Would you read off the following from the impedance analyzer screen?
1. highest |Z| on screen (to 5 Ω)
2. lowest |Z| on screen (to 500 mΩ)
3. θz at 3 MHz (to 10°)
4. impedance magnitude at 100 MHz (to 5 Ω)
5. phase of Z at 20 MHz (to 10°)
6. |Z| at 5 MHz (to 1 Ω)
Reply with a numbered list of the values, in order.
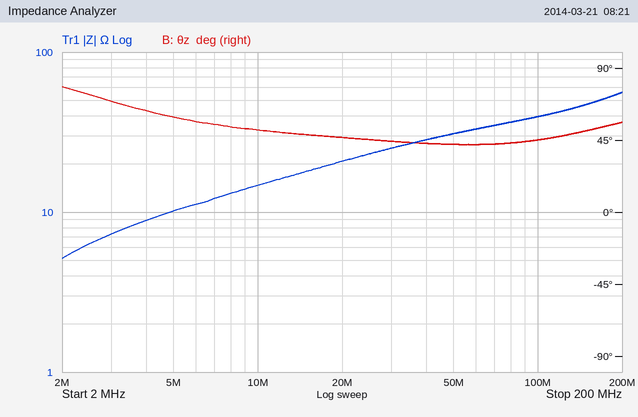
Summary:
1. 55 Ω
2. 5.0 Ω
3. 70°
4. 40 Ω
5. 50°
6. 10 Ω
